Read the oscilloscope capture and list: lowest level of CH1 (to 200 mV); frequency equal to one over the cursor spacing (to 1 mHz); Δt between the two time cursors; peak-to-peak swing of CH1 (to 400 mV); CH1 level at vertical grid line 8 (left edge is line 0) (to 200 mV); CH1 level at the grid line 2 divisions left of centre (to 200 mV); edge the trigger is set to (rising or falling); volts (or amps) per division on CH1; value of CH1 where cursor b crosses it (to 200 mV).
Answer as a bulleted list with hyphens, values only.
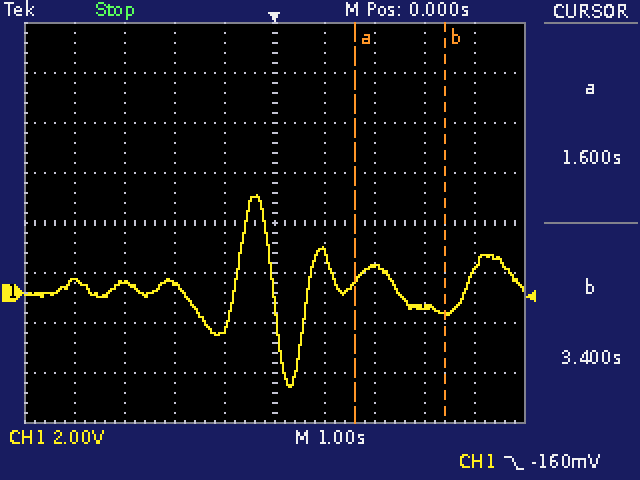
- -3.8 V
- 556 mHz
- 1.8 s
- 7.6 V
- -600 mV
- 400 mV
- falling
- 2 V
- -800 mV
